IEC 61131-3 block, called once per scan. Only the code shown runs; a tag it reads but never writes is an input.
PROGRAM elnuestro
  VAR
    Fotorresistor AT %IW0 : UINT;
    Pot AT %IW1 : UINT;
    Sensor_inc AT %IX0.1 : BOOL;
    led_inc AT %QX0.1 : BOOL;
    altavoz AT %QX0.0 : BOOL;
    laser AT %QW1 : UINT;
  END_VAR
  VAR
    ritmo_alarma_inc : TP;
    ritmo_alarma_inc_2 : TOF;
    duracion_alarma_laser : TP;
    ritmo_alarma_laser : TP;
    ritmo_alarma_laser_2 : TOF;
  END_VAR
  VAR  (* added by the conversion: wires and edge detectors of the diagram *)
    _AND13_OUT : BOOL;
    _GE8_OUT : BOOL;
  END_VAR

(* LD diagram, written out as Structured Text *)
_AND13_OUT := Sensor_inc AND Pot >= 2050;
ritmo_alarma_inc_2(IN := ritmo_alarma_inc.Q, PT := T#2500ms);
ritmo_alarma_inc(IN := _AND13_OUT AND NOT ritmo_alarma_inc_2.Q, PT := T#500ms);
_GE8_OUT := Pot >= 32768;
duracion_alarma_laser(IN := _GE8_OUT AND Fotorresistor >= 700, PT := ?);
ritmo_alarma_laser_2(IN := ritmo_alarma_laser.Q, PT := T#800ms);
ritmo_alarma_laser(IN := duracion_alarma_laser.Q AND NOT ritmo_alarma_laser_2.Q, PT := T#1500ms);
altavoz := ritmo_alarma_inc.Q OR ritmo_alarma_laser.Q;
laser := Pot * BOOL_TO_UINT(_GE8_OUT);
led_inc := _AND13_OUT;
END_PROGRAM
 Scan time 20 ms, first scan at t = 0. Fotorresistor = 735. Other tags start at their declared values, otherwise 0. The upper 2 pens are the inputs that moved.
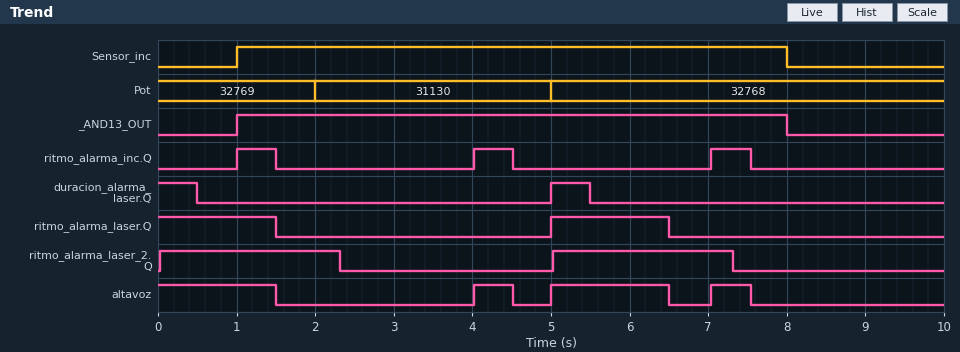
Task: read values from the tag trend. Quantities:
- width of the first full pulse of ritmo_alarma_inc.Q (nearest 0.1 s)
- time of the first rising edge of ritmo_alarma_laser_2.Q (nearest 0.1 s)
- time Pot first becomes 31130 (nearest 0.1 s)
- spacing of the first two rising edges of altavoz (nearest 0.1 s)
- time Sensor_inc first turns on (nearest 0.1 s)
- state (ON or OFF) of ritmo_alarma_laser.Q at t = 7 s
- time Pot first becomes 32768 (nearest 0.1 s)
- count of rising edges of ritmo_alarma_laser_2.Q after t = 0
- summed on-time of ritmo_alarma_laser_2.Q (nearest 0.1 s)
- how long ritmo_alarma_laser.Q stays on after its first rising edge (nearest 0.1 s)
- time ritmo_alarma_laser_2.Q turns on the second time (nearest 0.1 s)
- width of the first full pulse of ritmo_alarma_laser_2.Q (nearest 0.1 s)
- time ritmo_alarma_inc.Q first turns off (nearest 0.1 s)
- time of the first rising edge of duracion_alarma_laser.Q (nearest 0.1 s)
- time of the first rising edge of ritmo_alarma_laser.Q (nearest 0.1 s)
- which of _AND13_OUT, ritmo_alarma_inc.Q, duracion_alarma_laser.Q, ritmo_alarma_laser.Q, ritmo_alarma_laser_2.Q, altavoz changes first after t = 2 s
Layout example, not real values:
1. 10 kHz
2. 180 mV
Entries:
1. 0.5 s
2. 0.0 s
3. 2.0 s
4. 1.0 s
5. 1.0 s
6. OFF
7. 5.0 s
8. 2
9. 4.6 s
10. 1.5 s
11. 5.0 s
12. 2.3 s
13. 1.5 s
14. 5.0 s
15. 5.0 s
16. ritmo_alarma_laser_2.Q
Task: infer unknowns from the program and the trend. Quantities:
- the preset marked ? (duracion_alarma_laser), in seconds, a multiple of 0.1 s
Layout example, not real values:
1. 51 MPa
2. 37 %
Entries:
1. 0.5 s
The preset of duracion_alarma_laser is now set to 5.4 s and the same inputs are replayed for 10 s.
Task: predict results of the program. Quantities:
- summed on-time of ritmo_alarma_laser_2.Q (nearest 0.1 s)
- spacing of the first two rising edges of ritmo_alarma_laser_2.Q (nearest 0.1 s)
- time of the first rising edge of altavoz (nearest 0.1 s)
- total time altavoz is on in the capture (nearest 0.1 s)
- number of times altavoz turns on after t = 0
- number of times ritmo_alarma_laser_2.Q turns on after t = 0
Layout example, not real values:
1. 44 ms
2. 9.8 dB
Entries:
1. 6.9 s
2. 2.3 s
3. 2.3 s
4. 5.5 s
5. 4
6. 3
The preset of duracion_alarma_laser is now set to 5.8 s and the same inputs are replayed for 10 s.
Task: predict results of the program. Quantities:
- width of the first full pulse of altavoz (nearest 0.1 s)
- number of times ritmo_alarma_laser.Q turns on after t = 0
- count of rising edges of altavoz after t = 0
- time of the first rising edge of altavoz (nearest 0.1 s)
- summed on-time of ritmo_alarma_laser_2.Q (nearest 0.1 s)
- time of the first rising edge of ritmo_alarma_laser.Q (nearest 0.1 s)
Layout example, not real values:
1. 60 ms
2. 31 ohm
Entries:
1. 1.5 s
2. 2
3. 4
4. 2.3 s
5. 6.9 s
6. 2.3 s
